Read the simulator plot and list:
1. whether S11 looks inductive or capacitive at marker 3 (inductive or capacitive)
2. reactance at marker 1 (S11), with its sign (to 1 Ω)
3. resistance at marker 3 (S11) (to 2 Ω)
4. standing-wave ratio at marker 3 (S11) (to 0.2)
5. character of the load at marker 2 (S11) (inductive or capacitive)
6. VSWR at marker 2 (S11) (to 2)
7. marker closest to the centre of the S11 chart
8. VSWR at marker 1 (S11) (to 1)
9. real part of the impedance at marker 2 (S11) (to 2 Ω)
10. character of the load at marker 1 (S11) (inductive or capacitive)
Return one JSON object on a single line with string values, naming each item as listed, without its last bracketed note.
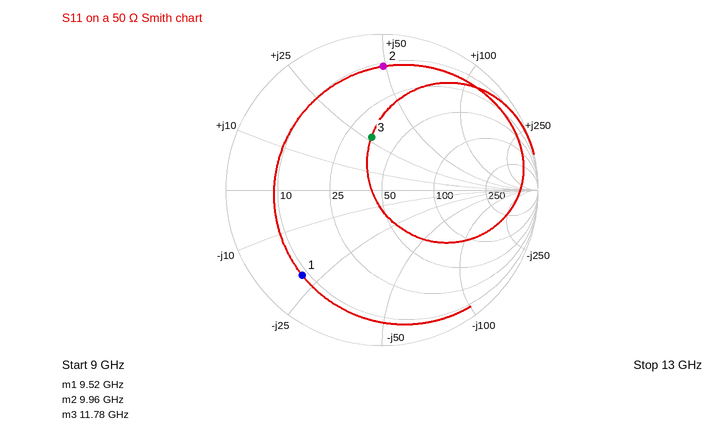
{"whether S11 looks inductive or capacitive at marker 3": "inductive", "reactance at marker 1 (S11), with its sign": "-21 Ω", "resistance at marker 3 (S11)": "36 Ω", "standing-wave ratio at marker 3 (S11)": "2.0", "character of the load at marker 2 (S11)": "inductive", "VSWR at marker 2 (S11)": "8", "marker closest to the centre of the S11 chart": "marker 3", "VSWR at marker 1 (S11)": "7", "real part of the impedance at marker 2 (S11)": "12 Ω", "character of the load at marker 1 (S11)": "capacitive"}
